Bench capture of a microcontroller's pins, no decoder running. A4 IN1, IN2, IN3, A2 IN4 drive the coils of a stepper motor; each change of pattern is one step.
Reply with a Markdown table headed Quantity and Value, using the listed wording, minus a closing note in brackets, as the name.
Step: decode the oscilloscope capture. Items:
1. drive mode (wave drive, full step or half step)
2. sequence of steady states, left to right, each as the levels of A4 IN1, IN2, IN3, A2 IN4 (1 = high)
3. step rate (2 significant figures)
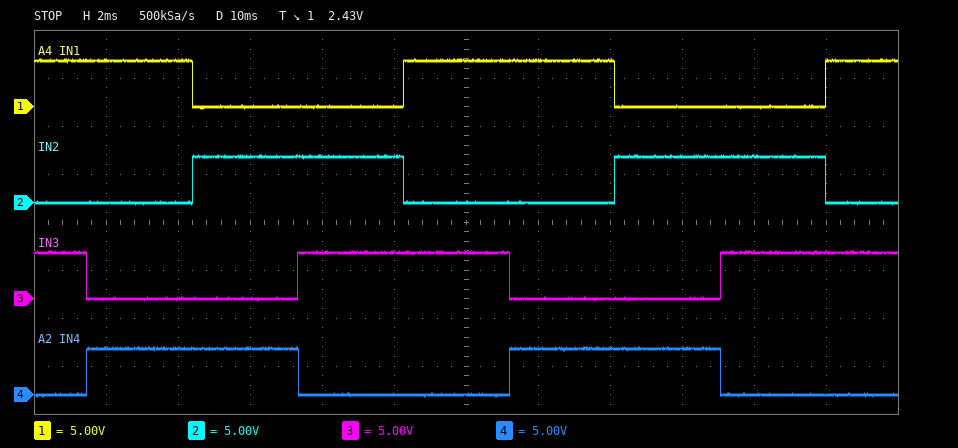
| Quantity | Value |
|---|---|
| drive mode | full step |
| sequence of steady states, left to right, each as the levels of A4 IN1, IN2, IN3, A2 IN4 | 1010 1001 0101 0110 1010 1001 0101 0110 1010 |
| step rate | 340 steps/s |
